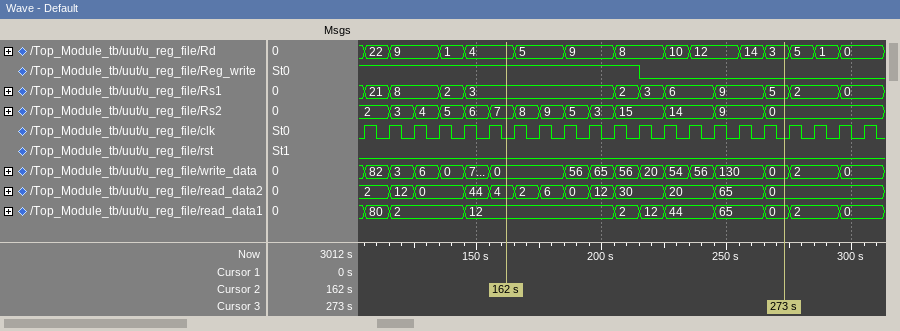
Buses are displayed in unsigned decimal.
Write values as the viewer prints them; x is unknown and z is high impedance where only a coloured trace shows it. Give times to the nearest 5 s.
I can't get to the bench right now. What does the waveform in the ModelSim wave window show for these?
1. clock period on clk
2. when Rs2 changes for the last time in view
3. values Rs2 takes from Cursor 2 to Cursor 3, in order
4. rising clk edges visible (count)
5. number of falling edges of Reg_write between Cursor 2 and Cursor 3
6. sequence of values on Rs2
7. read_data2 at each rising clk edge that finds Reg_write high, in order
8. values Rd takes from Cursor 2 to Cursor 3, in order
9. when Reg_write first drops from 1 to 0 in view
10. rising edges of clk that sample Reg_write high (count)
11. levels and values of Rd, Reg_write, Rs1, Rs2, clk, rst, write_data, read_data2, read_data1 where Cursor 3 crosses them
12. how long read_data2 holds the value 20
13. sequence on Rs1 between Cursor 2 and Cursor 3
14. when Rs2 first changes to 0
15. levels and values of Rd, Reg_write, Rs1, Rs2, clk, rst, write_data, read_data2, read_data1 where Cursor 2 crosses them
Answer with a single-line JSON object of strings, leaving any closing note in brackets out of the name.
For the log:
{"clock period on clk": "10 s", "when Rs2 changes for the last time in view": "265 s", "values Rs2 takes from Cursor 2 to Cursor 3, in order": "7, 8, 9, 5, 3, 15, 14, 9, 0", "rising clk edges visible": "21", "number of falling edges of Reg_write between Cursor 2 and Cursor 3": "1", "sequence of values on Rs2": "2, 3, 4, 5, 6, 7, 8, 9, 5, 3, 15, 14, 9, 0", "read_data2 at each rising clk edge that finds Reg_write high, in order": "2, 2, 12, 0, 0, 44, 4, 2, 6, 0, 12, 30", "values Rd takes from Cursor 2 to Cursor 3, in order": "4, 5, 9, 8, 10, 12, 14, 3", "when Reg_write first drops from 1 to 0 in view": "215 s", "rising edges of clk that sample Reg_write high": "12", "levels and values of Rd, Reg_write, Rs1, Rs2, clk, rst, write_data, read_data2, read_data1 where Cursor 3 crosses them": "Rd=3, Reg_write=0, Rs1=5, Rs2=0, clk=0, rst=0, write_data=0, read_data2=0, read_data1=0", "how long read_data2 holds the value 20": "20 s", "sequence on Rs1 between Cursor 2 and Cursor 3": "3, 2, 3, 6, 9, 5", "when Rs2 first changes to 0": "265 s", "levels and values of Rd, Reg_write, Rs1, Rs2, clk, rst, write_data, read_data2, read_data1 where Cursor 2 crosses them": "Rd=4, Reg_write=1, Rs1=3, Rs2=7, clk=0, rst=0, write_data=0, read_data2=4, read_data1=12"}
